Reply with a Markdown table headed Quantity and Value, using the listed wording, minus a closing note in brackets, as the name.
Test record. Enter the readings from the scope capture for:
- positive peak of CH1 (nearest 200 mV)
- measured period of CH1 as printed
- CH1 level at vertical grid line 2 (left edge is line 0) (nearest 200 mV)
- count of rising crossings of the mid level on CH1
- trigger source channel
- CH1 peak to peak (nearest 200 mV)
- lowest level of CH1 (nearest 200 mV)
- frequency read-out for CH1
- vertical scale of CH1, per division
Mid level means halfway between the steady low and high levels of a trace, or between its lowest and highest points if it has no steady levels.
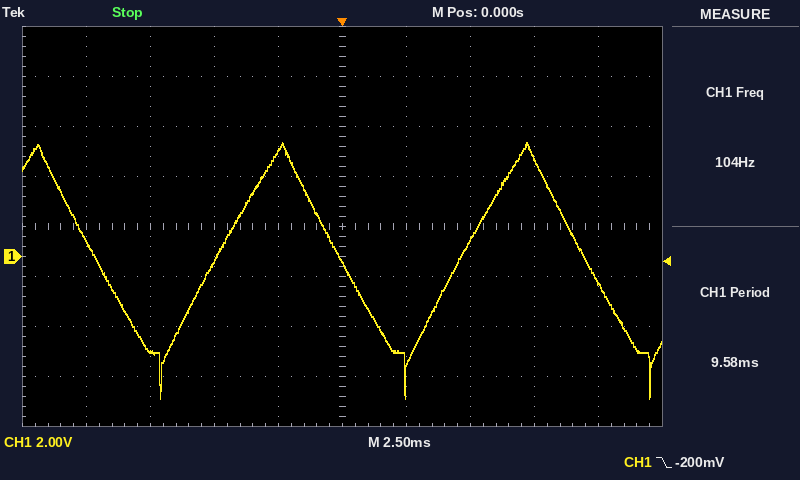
| Quantity | Value |
|---|---|
| positive peak of CH1 | 4.6 V |
| measured period of CH1 as printed | 9.58 ms |
| CH1 level at vertical grid line 2 (left edge is line 0) | -3.8 V |
| count of rising crossings of the mid level on CH1 | 2 |
| trigger source channel | CH1 |
| CH1 peak to peak | 10.2 V |
| lowest level of CH1 | -5.6 V |
| frequency read-out for CH1 | 104 Hz |
| vertical scale of CH1, per division | 2 V |
